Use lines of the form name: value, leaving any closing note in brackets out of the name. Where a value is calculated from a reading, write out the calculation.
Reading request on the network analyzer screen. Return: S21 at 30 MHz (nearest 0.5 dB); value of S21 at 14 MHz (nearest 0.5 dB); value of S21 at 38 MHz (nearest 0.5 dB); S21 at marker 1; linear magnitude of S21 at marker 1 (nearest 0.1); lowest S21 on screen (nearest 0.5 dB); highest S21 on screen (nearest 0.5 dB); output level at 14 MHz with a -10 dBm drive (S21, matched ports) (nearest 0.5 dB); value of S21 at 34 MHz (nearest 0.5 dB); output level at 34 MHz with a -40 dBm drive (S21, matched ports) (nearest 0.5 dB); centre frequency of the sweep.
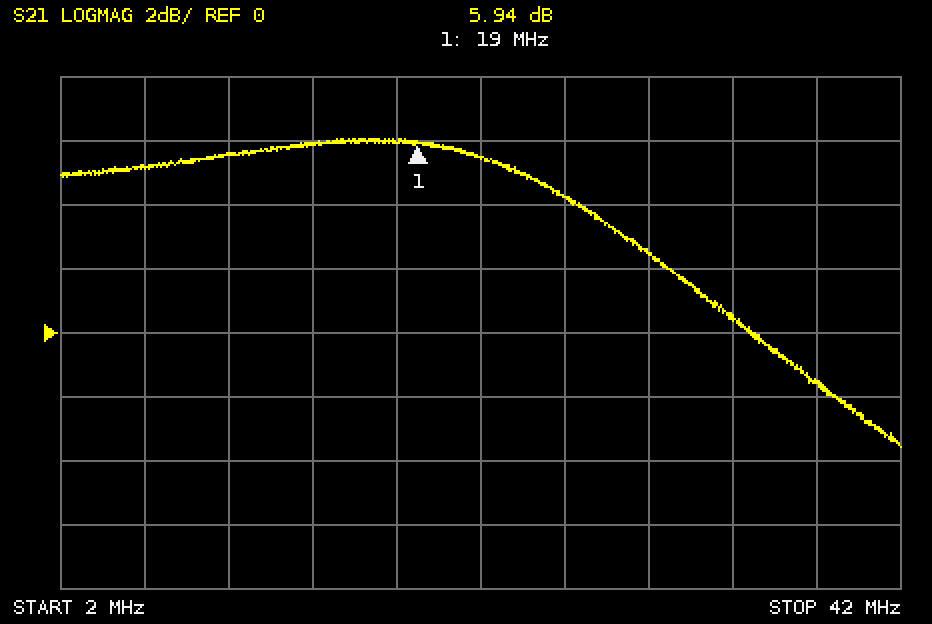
S21 at 30 MHz: 2.5 dB
value of S21 at 14 MHz: 6.0 dB
value of S21 at 38 MHz: -1.5 dB
S21 at marker 1: 5.94 dB
linear magnitude of S21 at marker 1: 10^(5.94/20) ≈ 2.0
lowest S21 on screen: -3.5 dB
highest S21 on screen: 6.0 dB
output level at 14 MHz with a -10 dBm drive (S21, matched ports): -10 dBm + (6.0 dB) = -4.0 dBm
value of S21 at 34 MHz: 0.5 dB
output level at 34 MHz with a -40 dBm drive (S21, matched ports): -40 dBm + (0.5 dB) = -39.5 dBm
centre frequency of the sweep: 22 MHz
